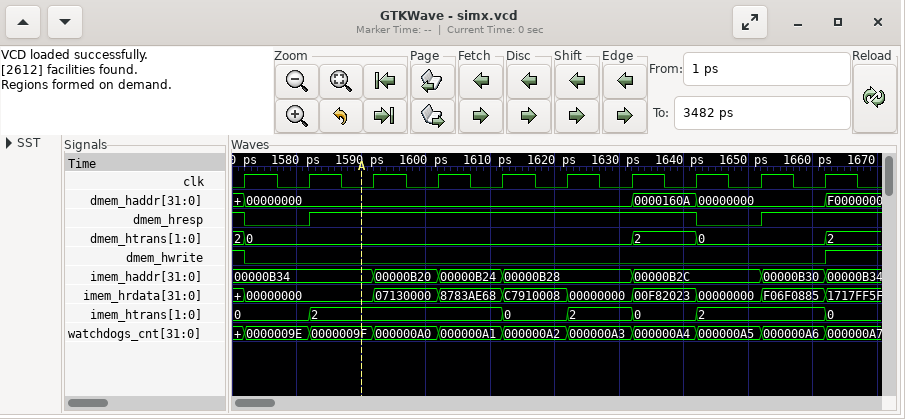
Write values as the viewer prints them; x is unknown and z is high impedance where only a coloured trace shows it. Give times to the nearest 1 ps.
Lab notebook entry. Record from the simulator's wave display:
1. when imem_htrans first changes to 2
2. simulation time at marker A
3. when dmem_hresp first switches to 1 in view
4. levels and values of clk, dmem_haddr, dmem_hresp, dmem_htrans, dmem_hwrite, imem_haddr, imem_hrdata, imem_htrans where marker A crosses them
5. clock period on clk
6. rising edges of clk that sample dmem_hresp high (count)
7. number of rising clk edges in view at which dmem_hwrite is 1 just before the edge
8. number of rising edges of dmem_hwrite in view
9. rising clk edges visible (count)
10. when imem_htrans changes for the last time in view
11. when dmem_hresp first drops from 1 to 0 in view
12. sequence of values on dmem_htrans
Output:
1582 ps
1590 ps
1582 ps
clk=0, dmem_haddr=00000000, dmem_hresp=1, dmem_htrans=0, dmem_hwrite=0, imem_haddr=00000B34, imem_hrdata=00000000, imem_htrans=2
10 ps
8
1
1
10
1662 ps
1572 ps
2, 0, 2, 0, 2
